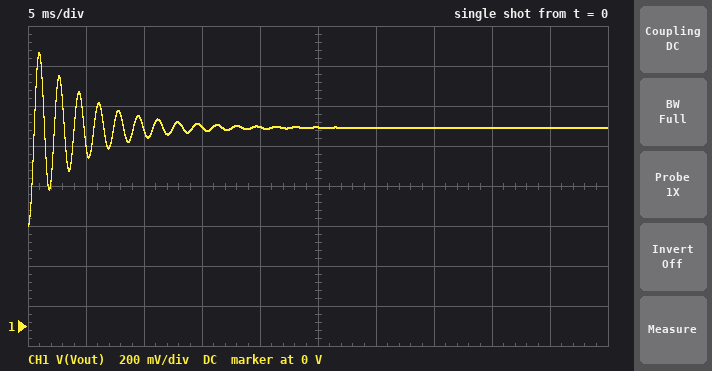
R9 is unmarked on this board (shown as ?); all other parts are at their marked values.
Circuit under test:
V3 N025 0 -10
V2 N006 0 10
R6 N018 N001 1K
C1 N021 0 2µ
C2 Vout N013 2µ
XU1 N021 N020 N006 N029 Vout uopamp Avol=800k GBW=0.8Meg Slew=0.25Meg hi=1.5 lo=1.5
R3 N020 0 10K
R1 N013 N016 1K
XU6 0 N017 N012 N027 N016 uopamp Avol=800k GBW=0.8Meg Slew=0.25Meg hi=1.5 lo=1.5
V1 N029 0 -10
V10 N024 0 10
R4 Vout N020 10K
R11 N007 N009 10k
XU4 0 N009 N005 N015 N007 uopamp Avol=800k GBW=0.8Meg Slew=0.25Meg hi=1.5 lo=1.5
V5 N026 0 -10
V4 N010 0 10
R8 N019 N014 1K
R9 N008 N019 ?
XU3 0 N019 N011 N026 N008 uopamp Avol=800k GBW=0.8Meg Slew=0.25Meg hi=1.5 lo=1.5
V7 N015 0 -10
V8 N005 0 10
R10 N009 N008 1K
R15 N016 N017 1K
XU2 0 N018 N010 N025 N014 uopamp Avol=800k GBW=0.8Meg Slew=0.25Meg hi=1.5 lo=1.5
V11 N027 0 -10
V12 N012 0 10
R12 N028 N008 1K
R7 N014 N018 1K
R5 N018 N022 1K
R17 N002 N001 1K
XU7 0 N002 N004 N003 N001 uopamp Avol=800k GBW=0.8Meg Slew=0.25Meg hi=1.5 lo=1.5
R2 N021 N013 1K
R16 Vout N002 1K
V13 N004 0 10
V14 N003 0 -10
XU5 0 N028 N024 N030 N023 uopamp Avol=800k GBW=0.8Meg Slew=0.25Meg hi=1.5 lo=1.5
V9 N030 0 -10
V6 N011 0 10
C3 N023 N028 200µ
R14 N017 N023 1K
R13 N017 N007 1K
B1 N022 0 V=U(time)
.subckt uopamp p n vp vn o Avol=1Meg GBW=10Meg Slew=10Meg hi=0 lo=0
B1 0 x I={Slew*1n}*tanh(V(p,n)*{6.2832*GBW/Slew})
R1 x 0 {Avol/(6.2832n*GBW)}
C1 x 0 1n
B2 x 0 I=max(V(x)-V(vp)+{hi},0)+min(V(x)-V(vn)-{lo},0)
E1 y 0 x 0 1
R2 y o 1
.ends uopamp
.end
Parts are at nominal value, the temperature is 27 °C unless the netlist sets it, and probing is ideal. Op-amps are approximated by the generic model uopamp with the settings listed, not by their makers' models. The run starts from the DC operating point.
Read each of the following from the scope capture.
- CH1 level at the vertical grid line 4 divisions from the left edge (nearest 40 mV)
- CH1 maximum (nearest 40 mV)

1.00 V
1.36 V
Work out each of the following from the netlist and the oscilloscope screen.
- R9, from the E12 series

2.7 kΩ
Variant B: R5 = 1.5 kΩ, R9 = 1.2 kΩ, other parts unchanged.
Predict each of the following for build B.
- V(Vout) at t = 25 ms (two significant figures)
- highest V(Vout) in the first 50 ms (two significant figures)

650 mV
890 mV
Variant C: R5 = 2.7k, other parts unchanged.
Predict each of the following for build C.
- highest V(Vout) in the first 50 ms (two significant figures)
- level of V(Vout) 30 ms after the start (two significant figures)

520 mV
370 mV
